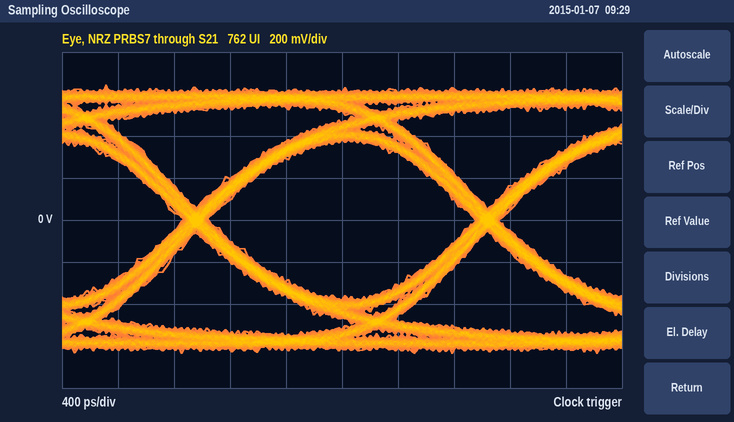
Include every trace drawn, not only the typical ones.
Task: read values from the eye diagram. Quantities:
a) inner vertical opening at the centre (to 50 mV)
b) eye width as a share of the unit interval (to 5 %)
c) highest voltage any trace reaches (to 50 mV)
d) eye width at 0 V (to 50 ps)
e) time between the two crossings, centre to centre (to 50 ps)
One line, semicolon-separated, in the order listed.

750 mV; 90 %; 650 mV; 1.90 ns; 2.10 ns
